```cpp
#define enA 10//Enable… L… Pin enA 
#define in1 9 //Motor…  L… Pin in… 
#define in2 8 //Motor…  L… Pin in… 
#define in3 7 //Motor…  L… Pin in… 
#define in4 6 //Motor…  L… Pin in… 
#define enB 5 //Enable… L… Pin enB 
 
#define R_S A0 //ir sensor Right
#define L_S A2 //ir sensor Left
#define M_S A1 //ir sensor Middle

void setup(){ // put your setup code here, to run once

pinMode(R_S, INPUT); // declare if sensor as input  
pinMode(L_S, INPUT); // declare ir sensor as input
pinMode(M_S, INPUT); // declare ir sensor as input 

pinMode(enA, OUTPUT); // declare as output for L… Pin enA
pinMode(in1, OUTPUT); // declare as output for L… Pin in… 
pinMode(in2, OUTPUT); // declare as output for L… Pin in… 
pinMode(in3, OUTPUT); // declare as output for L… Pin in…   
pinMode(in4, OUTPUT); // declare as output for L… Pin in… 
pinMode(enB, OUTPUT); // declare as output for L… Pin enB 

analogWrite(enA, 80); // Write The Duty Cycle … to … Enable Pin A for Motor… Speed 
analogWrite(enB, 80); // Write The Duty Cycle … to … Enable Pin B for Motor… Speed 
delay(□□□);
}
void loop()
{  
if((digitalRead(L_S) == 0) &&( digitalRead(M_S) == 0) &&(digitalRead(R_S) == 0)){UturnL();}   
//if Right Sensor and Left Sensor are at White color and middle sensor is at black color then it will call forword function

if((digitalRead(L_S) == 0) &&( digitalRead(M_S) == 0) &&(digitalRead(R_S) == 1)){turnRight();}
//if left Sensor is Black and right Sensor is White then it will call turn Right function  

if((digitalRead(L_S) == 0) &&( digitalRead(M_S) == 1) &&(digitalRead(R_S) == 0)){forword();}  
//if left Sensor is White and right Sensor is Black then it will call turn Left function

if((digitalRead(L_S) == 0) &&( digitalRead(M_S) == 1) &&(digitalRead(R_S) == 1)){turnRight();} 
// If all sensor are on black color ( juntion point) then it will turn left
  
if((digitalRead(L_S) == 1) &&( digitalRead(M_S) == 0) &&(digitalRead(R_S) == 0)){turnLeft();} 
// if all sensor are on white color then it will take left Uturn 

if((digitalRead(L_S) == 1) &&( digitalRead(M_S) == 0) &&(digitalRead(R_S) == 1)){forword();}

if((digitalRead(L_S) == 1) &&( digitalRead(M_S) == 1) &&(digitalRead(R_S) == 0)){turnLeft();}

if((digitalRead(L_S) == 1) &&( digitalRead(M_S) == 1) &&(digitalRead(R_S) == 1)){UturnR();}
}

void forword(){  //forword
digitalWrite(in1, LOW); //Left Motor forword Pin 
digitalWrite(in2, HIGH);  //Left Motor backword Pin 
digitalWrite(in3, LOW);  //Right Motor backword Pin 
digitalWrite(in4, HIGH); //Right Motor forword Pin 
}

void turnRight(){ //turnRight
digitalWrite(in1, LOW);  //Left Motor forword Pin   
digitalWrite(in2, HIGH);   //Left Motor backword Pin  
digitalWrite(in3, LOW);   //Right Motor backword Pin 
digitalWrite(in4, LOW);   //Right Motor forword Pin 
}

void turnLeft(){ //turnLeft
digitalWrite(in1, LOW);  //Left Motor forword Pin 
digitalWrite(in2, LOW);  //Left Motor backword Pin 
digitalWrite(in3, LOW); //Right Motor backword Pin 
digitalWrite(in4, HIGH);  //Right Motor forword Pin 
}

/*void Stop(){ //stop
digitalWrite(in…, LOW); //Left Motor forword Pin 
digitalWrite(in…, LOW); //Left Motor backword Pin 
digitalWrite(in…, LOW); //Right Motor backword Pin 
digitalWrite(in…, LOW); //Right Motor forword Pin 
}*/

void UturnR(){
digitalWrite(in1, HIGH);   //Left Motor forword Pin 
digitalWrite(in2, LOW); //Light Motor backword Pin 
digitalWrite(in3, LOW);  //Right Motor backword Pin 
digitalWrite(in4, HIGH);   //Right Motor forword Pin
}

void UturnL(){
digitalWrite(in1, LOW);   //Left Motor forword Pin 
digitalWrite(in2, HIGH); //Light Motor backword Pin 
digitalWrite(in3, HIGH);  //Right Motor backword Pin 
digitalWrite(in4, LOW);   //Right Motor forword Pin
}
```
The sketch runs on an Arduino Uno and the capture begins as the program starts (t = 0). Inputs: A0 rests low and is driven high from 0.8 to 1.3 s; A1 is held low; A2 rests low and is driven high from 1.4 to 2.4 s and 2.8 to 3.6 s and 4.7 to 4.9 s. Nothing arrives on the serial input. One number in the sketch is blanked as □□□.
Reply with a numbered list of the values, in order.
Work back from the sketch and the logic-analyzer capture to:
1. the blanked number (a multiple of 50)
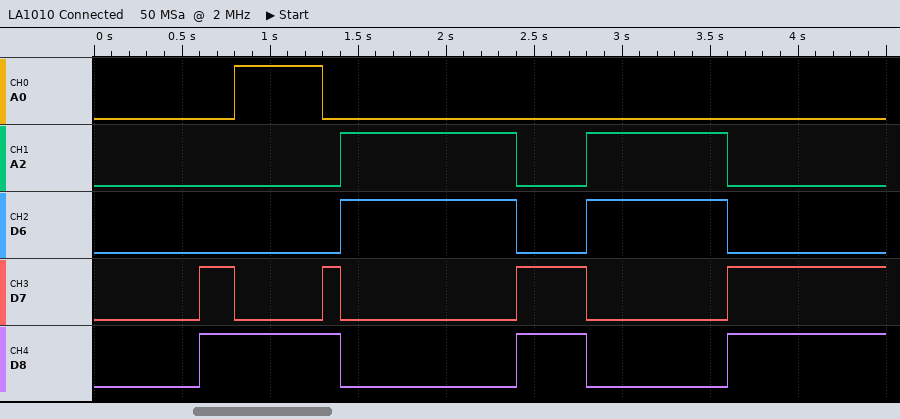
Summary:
1. 600
